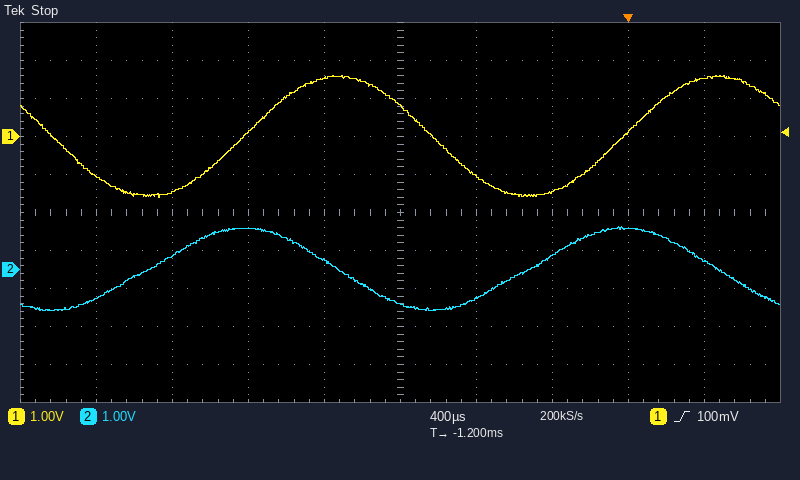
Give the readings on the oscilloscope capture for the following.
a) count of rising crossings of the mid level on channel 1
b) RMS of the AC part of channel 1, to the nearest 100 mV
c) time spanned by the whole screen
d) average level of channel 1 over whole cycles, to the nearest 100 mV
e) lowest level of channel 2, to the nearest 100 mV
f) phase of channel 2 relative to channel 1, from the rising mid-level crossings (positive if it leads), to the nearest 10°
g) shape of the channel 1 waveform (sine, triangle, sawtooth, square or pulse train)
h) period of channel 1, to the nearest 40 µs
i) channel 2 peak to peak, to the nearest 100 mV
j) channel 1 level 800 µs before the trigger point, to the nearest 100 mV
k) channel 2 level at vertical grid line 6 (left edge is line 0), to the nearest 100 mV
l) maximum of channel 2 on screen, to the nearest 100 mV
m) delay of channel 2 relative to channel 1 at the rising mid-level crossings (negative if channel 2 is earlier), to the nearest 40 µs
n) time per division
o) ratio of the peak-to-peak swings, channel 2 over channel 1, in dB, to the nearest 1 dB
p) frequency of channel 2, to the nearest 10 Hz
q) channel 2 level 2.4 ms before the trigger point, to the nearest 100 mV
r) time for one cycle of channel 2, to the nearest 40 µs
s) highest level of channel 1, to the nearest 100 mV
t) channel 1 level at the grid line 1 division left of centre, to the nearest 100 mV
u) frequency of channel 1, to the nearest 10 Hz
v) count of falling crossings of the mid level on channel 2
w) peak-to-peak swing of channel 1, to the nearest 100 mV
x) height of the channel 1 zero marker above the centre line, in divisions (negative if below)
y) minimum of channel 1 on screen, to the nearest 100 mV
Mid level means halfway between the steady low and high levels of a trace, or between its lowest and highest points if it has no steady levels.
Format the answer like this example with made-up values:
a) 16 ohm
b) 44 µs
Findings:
a) 2
b) 1.1 V
c) 4 ms
d) 0.0 V
e) -1.1 V
f) +90°
g) sine
h) 2.00 ms
i) 2.2 V
j) -1.0 V
k) -800 mV
l) 1.1 V
m) -480 µs
n) 400 µs
o) -3 dB
p) 500 Hz
q) 400 mV
r) 2.00 ms
s) 1.6 V
t) 1.5 V
u) 500 Hz
v) 2
w) 3.2 V
x) +2.0 div
y) -1.6 V
